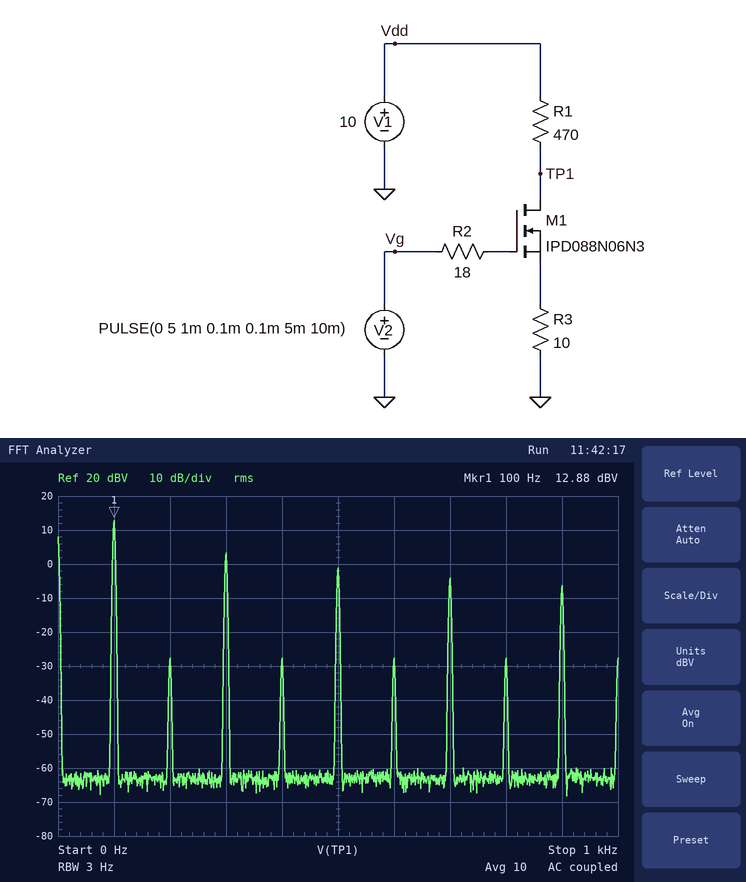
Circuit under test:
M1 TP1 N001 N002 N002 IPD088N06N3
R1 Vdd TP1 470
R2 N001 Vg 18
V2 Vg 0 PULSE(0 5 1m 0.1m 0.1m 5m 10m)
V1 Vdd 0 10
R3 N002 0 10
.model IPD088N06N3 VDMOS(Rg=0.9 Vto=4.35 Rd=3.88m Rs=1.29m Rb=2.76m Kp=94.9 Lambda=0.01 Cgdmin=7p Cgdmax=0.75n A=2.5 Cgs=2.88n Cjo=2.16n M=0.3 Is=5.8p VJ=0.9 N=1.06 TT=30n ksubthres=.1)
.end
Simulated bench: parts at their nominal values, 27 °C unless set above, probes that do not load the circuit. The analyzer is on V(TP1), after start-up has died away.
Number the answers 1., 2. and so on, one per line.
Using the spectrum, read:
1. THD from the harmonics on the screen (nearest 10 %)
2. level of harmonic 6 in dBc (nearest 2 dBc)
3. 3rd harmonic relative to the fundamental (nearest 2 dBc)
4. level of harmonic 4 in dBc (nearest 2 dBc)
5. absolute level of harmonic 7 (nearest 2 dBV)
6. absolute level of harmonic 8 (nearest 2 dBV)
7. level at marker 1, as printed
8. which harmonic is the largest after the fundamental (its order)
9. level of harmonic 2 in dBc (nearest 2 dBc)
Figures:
1. 40 %
2. -40 dBc
3. -10 dBc
4. -40 dBc
5. -4 dBV
6. -28 dBV
7. 12.88 dBV
8. 3
9. -40 dBc
